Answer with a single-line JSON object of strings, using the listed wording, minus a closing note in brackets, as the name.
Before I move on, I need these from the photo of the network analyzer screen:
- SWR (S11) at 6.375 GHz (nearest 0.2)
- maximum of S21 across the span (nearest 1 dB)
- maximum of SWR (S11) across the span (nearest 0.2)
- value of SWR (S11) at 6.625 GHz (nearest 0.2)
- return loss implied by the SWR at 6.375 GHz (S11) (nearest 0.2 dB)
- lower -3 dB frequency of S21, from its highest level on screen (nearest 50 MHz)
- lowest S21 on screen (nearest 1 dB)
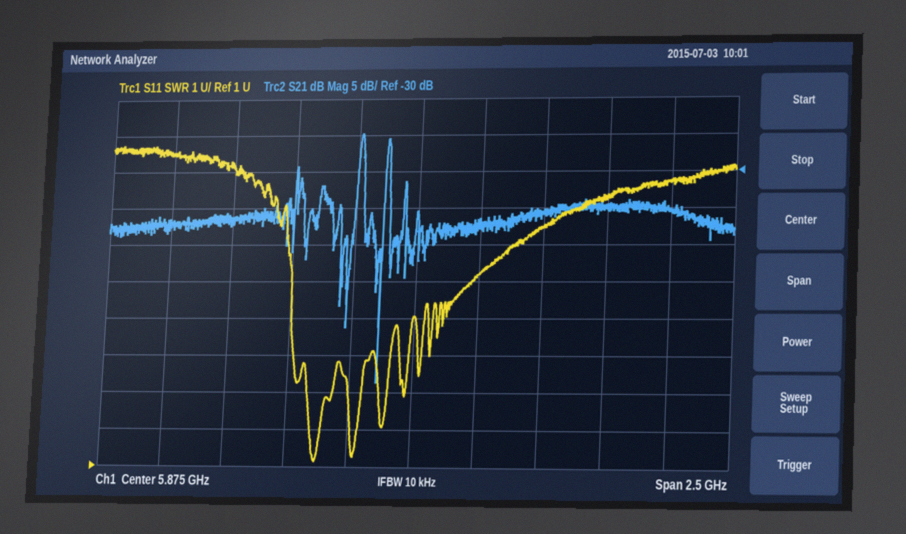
{"SWR (S11) at 6.375 GHz": "7.4", "maximum of S21 across the span": "-25 dB", "maximum of SWR (S11) across the span": "9.8", "value of SWR (S11) at 6.625 GHz": "8.2", "return loss implied by the SWR at 6.375 GHz (S11)": "2.4 dB", "lower -3 dB frequency of S21, from its highest level on screen": "5.65 GHz", "lowest S21 on screen": "-59 dB"}
